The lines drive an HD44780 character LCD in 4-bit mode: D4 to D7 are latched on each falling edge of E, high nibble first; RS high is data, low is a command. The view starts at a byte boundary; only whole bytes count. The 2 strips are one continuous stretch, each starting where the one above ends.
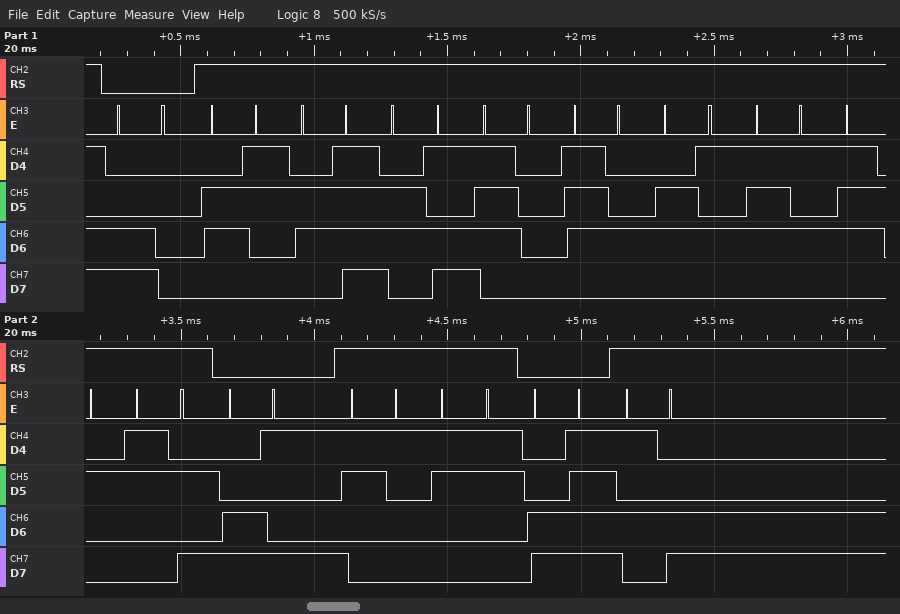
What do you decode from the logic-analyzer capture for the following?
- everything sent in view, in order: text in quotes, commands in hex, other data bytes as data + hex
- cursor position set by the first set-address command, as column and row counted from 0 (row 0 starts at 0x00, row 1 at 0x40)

0xC0 "compteur:" 0xC9 "13" 0xCF data 5C
column 0, row 1
